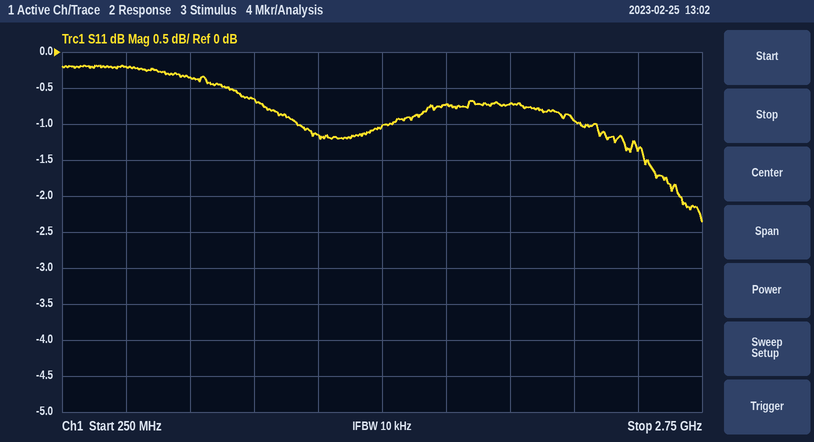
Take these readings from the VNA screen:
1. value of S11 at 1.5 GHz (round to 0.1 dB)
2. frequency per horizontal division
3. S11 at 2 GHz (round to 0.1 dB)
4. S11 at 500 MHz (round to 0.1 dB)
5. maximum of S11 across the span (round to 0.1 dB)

-1.0 dB
250 MHz
-0.7 dB
-0.2 dB
-0.2 dB
